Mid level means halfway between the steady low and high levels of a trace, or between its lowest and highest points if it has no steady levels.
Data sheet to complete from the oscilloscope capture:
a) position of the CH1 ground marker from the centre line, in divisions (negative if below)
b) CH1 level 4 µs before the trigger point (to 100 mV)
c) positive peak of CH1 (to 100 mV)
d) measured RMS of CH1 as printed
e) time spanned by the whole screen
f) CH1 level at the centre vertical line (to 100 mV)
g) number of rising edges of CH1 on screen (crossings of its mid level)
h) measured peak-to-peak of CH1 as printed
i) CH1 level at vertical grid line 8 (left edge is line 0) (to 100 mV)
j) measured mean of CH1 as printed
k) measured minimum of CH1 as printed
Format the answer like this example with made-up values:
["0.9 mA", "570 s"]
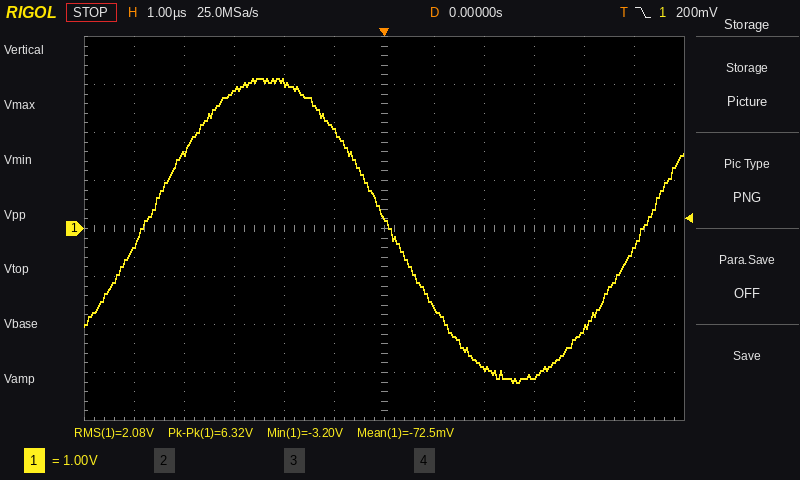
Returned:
["0.0 div", "1.6 V", "3.1 V", "2.08 V", "12 µs", "200 mV", "2", "6.32 V", "-2.9 V", "-72.5 mV", "-3.20 V"]
